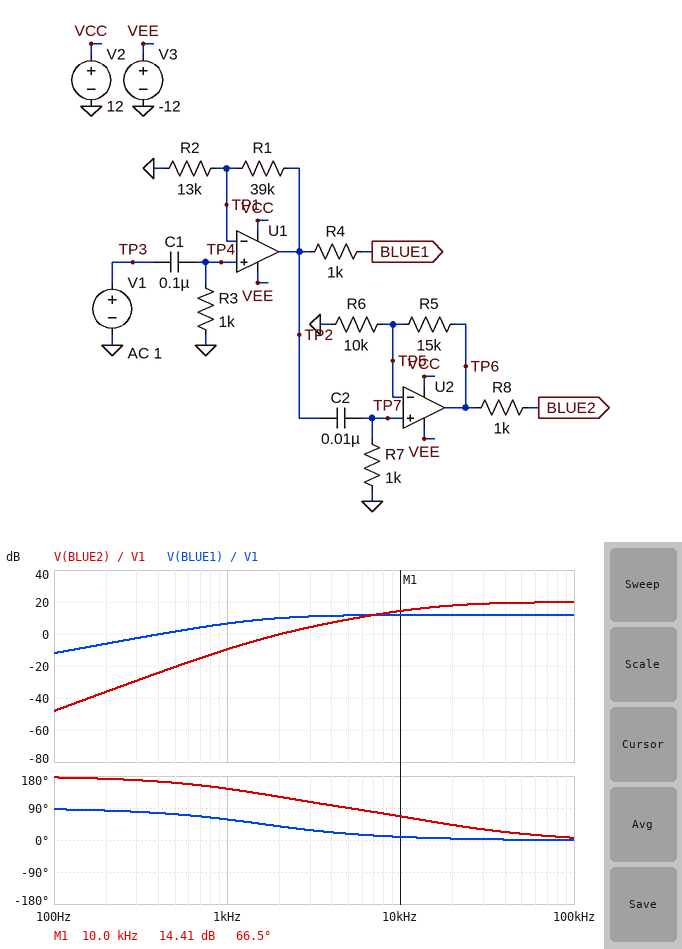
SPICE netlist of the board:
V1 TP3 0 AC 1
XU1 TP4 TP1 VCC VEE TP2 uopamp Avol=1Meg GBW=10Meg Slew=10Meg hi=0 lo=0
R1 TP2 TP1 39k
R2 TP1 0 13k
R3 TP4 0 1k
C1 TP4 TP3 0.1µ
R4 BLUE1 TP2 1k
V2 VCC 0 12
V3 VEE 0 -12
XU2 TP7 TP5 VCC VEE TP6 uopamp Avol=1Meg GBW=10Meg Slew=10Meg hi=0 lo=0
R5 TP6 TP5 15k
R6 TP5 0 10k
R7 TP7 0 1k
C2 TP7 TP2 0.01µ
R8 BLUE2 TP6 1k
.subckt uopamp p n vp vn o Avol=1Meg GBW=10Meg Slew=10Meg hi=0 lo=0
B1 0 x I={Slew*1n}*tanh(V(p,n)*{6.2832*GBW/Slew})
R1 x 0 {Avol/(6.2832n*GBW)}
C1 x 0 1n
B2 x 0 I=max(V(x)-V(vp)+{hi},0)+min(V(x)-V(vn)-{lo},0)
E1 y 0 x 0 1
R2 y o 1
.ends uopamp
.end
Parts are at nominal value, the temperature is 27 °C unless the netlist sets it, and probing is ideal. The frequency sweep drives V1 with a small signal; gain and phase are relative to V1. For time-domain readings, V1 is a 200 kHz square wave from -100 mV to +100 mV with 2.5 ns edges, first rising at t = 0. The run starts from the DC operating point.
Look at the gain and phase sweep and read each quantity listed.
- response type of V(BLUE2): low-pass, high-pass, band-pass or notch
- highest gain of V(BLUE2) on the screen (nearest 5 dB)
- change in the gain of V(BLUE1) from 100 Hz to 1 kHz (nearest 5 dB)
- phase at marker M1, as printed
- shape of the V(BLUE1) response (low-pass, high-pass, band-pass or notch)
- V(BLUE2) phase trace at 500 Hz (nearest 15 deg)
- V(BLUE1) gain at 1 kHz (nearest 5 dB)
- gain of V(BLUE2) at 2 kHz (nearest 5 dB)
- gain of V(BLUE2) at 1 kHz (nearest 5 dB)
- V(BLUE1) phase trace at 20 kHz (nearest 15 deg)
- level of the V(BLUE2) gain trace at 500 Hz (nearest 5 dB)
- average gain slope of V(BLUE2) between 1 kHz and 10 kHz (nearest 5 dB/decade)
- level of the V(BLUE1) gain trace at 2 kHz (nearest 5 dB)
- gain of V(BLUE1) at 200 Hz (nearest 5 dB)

high-pass
20 dB
20 dB
66.5 deg
high-pass
165 deg
5 dB
0 dB
-10 dB
0 deg
-20 dB
25 dB/decade
10 dB
-5 dB
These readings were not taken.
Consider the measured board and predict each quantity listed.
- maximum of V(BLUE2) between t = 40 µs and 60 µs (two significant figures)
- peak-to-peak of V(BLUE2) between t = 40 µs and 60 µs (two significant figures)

1.0 V
2.2 V
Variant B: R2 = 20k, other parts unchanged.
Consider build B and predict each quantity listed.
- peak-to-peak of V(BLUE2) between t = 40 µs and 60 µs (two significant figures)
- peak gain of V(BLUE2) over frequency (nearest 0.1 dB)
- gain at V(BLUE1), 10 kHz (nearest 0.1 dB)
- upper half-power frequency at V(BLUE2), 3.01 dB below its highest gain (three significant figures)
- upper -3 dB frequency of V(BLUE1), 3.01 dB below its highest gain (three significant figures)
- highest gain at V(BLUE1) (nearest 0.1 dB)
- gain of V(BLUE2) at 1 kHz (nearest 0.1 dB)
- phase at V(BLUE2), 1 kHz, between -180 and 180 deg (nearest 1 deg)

1.6 V
17.3 dB
9.3 dB
2.38 MHz
3.39 MHz
9.4 dB
-12.2 dB
144 deg
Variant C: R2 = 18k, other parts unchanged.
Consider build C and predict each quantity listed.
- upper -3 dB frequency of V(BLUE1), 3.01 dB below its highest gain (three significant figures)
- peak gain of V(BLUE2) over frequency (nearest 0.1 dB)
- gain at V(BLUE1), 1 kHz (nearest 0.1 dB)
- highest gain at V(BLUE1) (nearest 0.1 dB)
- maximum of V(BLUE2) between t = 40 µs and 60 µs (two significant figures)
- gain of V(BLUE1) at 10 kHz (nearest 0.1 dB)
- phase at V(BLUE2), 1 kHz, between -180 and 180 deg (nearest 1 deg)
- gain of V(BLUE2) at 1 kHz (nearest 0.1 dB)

3.16 MHz
17.9 dB
4.5 dB
10.0 dB
820 mV
9.9 dB
144 deg
-11.6 dB
